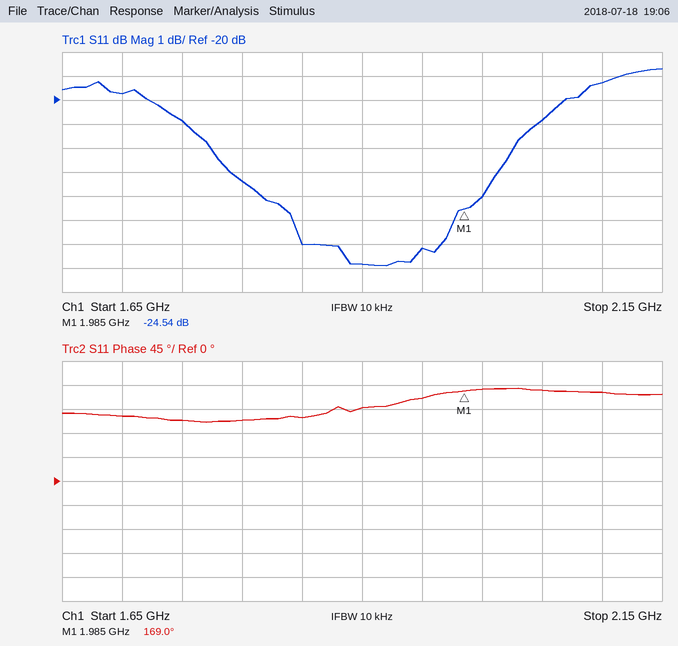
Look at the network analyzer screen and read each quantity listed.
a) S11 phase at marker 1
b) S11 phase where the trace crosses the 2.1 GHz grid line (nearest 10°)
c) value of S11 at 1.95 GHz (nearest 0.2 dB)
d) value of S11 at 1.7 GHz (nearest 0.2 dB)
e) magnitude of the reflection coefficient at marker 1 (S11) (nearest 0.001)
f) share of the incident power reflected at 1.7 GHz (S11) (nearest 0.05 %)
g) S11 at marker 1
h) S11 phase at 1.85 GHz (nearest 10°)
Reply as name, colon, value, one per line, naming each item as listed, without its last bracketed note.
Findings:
S11 phase at marker 1: 169.0°
S11 phase where the trace crosses the 2.1 GHz grid line: 170°
value of S11 at 1.95 GHz: -26.2 dB
value of S11 at 1.7 GHz: -19.8 dB
magnitude of the reflection coefficient at marker 1 (S11): 0.059
share of the incident power reflected at 1.7 GHz (S11): 1.05 %
S11 at marker 1: -24.54 dB
S11 phase at 1.85 GHz: 120°
